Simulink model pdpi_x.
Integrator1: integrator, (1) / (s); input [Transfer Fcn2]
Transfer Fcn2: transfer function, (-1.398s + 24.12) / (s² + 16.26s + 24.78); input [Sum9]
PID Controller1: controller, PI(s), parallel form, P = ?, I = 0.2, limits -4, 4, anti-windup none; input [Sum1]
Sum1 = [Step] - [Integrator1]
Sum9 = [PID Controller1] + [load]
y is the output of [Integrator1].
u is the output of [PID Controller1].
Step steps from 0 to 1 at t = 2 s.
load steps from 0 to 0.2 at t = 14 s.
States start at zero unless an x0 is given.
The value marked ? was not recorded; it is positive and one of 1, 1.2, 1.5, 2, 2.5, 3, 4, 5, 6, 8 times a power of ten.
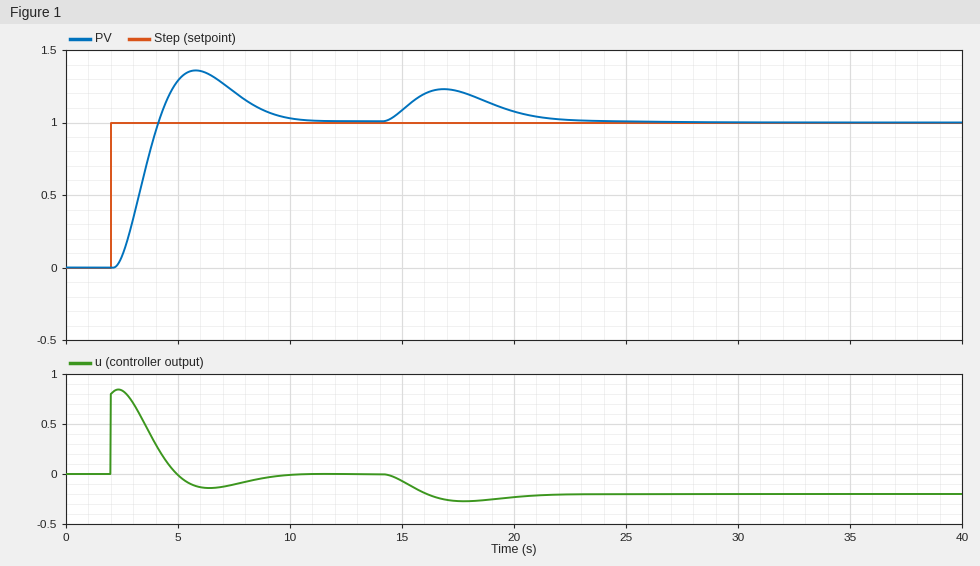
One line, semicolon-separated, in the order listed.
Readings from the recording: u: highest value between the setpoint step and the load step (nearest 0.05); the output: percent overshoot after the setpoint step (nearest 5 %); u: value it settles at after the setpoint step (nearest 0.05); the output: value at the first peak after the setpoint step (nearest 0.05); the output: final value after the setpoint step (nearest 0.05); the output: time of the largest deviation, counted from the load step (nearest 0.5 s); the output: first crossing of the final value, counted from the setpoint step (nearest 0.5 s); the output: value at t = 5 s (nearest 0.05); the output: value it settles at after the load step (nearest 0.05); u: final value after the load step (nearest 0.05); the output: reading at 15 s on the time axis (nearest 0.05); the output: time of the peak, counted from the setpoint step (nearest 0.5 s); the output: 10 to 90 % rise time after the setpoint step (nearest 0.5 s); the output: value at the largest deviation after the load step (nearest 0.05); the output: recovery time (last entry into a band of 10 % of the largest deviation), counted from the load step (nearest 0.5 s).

0.85; 35 %; 0.00; 1.35; 1.00; 3.0 s; 2.0 s; 1.30; 1.00; -0.20; 1.10; 4.0 s; 1.5 s; 1.25; 8.0 s
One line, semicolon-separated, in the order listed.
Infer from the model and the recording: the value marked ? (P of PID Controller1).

0.8
